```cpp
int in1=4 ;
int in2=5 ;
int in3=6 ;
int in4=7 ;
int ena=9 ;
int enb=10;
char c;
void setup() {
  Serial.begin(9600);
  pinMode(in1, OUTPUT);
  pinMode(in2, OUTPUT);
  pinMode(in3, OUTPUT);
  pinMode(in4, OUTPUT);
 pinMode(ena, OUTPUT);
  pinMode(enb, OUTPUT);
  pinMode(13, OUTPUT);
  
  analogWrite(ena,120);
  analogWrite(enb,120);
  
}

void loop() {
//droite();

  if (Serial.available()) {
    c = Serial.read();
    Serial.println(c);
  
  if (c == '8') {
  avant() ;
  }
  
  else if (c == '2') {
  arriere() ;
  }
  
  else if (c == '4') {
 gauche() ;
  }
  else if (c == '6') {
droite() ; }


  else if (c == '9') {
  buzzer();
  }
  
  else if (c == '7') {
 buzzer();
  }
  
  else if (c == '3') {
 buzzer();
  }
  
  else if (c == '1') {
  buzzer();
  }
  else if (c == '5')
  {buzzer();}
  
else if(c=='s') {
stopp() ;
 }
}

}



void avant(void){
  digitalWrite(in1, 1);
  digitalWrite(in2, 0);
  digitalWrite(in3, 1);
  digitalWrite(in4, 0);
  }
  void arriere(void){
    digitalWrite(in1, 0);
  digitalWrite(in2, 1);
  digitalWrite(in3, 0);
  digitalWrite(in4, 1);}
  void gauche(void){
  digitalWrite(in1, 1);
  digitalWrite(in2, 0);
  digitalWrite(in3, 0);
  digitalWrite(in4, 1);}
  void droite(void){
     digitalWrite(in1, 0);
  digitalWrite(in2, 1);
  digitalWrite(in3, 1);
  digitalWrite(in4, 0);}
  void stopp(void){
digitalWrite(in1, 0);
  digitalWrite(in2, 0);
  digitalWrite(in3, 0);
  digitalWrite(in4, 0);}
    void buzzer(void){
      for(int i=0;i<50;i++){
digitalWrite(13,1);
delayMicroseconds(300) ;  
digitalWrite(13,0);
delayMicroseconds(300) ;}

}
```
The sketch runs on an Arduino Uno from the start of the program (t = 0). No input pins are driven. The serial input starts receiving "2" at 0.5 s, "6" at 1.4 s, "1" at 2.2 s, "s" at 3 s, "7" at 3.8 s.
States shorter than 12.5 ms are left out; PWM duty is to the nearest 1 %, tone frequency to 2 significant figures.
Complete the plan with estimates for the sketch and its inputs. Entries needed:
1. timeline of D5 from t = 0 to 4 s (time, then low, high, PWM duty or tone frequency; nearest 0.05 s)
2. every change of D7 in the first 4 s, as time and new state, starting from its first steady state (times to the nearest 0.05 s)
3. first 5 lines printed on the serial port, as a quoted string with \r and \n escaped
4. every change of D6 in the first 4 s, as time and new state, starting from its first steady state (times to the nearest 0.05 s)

0 s low; 0.5 s high; 3 s low
0 s low; 0.5 s high; 1.4 s low
"2\r\n6\r\n1\r\ns\r\n7\r\n"
0 s low; 1.4 s high; 3 s low
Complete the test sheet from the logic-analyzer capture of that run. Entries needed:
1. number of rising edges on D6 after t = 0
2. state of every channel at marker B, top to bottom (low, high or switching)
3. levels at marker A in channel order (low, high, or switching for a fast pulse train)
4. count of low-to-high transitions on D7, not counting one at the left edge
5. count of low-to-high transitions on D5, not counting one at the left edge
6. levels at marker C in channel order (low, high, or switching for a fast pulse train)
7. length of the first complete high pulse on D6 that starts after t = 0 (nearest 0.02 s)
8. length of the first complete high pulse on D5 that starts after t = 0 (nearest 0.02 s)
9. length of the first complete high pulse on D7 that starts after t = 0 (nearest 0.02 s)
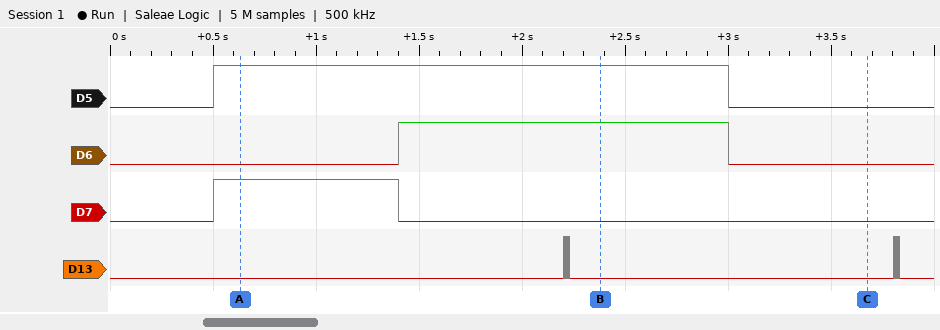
1
D5 high, D6 high, D7 low, D13 low
D5 high, D6 low, D7 high, D13 low
1
1
D5 low, D6 low, D7 low, D13 low
1.60 s
2.50 s
0.90 s
